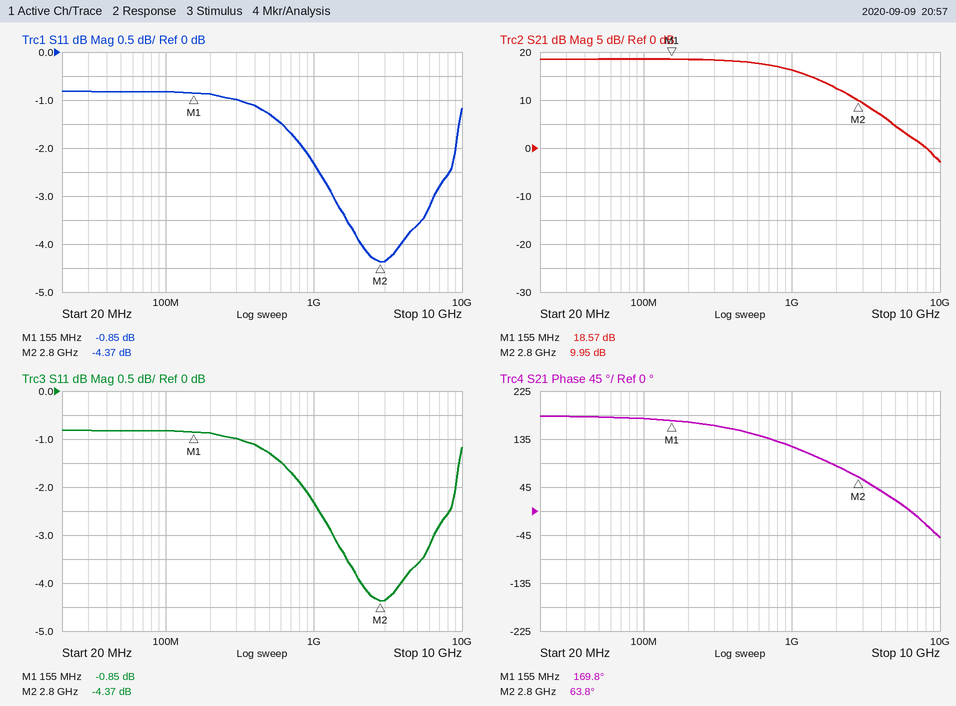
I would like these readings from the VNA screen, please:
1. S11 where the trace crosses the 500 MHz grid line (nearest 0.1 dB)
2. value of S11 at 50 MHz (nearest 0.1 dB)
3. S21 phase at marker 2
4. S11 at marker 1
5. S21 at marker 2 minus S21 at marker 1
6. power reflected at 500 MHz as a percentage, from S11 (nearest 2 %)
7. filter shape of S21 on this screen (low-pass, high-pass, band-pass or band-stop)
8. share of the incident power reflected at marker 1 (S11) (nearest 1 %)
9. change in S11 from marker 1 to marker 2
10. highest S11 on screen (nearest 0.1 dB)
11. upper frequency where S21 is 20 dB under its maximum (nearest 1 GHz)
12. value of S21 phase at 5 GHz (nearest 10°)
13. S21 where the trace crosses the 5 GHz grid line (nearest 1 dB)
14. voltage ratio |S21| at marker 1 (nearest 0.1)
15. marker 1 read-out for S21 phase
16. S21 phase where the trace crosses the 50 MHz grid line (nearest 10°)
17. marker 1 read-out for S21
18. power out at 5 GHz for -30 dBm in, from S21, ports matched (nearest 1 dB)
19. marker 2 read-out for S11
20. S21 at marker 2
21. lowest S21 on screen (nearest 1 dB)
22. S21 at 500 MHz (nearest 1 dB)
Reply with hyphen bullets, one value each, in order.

- -1.3 dB
- -0.8 dB
- 63.8°
- -0.85 dB
- -8.62 dB
- 74 %
- low-pass
- 82 %
- -3.52 dB
- -0.8 dB
- 9 GHz
- 20°
- 5 dB
- 8.5
- 169.8°
- 180°
- 18.57 dB
- -25 dBm
- -4.37 dB
- 9.95 dB
- -3 dB
- 18 dB
